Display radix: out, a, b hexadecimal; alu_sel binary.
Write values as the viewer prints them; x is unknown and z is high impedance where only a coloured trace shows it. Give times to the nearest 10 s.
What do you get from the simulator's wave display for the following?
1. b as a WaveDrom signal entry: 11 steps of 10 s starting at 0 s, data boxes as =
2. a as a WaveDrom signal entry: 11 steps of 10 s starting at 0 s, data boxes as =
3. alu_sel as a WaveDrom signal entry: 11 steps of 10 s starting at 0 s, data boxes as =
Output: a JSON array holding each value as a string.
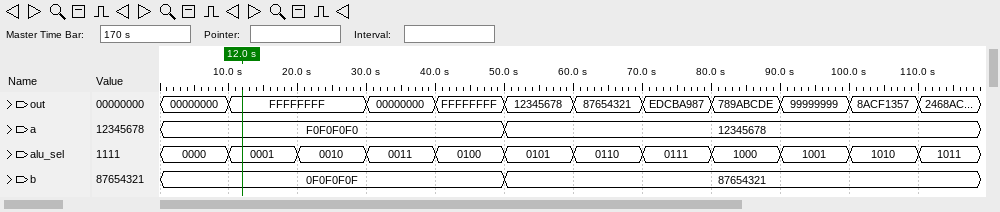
["{name: 'b', wave: '=....=.....', data: '0F0F0F0F 87654321'}", "{name: 'a', wave: '=....=.....', data: 'F0F0F0F0 12345678'}", "{name: 'alu_sel', wave: '===========', data: '0000 0001 0010 0011 0100 0101 0110 0111 1000 1001 1010'}"]
